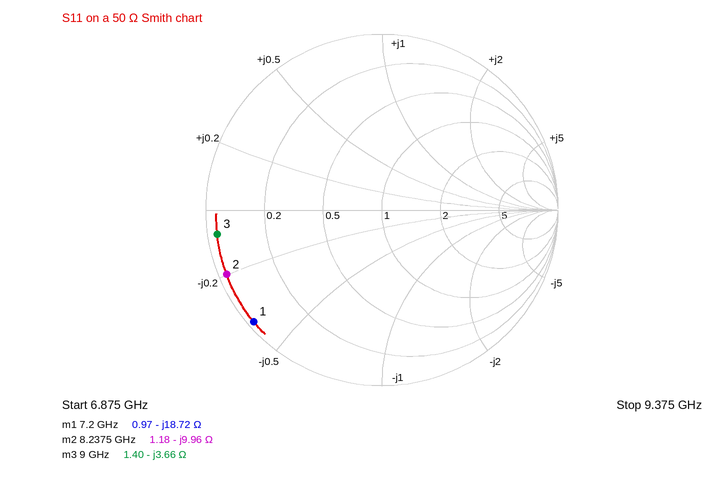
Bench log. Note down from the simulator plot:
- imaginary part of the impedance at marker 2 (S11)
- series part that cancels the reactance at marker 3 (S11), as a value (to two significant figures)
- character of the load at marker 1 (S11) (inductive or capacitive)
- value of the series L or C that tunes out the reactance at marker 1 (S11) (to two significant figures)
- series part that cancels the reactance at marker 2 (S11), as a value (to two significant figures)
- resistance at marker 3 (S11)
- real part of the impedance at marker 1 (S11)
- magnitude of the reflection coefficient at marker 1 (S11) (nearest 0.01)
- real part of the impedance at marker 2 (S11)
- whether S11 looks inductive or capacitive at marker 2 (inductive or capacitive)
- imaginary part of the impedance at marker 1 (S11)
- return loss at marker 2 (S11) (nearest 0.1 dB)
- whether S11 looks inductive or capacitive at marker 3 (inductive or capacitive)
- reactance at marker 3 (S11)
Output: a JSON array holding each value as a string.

["-9.96 Ω", "65 pH", "capacitive", "410 pH", "190 pH", "1.40 Ω", "0.97 Ω", "0.97", "1.18 Ω", "capacitive", "-18.72 Ω", "0.4 dB", "capacitive", "-3.66 Ω"]
